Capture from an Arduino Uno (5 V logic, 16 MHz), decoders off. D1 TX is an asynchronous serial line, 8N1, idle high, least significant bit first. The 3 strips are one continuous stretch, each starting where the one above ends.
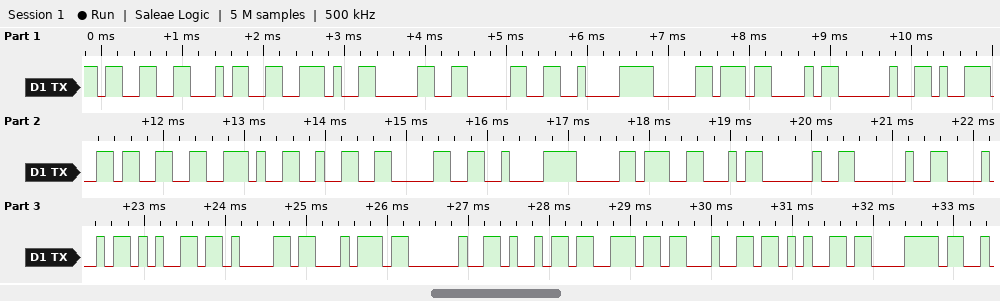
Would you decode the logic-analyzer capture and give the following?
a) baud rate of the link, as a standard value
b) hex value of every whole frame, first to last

9600 baud
33 34 2E 30 30 C2 B0 43 20 39 33 2E 32 30 C2 B0 46 20 20 48 65 61 74 20 69 6E 64 65 78
